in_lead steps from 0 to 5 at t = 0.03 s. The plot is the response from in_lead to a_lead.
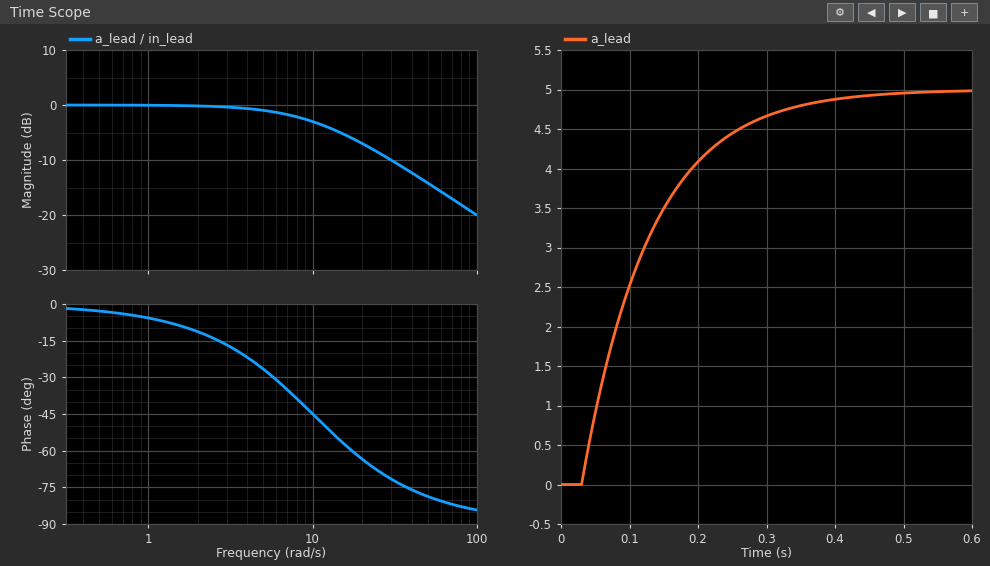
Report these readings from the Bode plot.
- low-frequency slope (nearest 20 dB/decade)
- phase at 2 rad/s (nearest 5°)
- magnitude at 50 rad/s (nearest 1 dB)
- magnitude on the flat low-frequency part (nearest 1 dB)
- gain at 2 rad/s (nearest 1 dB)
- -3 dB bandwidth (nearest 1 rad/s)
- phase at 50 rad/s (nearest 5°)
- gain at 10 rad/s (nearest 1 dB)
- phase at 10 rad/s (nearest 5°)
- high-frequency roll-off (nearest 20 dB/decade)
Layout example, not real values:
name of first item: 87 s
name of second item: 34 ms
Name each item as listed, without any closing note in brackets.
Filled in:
low-frequency slope: 0 dB/decade
phase at 2 rad/s: -10°
magnitude at 50 rad/s: -14 dB
magnitude on the flat low-frequency part: 0 dB
gain at 2 rad/s: 0 dB
-3 dB bandwidth: 10 rad/s
phase at 50 rad/s: -80°
gain at 10 rad/s: -3 dB
phase at 10 rad/s: -45°
high-frequency roll-off: -20 dB/decade
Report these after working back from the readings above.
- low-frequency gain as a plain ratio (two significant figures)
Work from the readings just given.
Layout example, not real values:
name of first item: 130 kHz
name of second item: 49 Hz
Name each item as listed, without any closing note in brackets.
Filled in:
low-frequency gain as a plain ratio: 1.0
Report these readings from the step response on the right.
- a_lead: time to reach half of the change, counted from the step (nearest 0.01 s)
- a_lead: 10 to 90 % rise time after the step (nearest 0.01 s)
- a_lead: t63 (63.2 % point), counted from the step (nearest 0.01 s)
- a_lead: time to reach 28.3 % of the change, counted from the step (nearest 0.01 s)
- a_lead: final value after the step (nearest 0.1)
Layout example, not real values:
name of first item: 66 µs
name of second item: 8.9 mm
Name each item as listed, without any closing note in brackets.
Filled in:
a_lead: time to reach half of the change, counted from the step: 0.07 s
a_lead: 10 to 90 % rise time after the step: 0.22 s
a_lead: t63 (63.2 % point), counted from the step: 0.10 s
a_lead: time to reach 28.3 % of the change, counted from the step: 0.03 s
a_lead: final value after the step: 5.0
